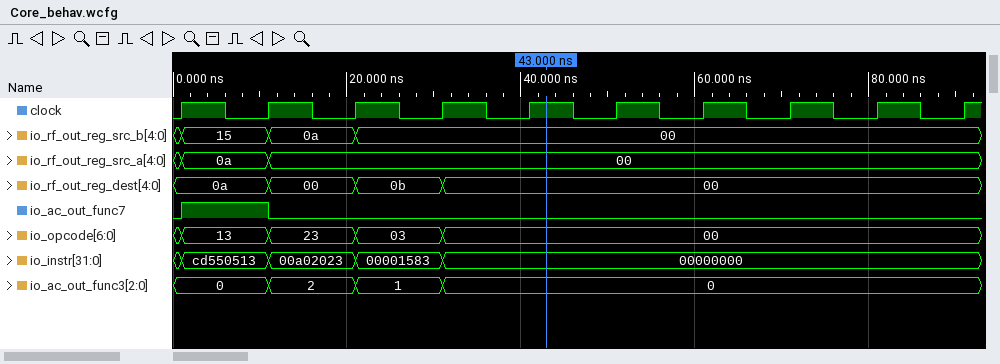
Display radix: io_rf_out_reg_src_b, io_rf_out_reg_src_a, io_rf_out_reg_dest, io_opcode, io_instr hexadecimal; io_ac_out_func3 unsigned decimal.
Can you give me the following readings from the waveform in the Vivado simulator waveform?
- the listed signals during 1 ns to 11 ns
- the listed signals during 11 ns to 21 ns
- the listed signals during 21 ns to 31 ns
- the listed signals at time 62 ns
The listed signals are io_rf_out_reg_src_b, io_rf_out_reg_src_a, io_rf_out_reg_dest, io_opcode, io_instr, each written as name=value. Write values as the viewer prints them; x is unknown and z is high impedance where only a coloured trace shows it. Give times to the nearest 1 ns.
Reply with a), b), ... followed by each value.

a) io_rf_out_reg_src_b=15, io_rf_out_reg_src_a=0a, io_rf_out_reg_dest=0a, io_opcode=13, io_instr=cd550513
b) io_rf_out_reg_src_b=0a, io_rf_out_reg_src_a=00, io_rf_out_reg_dest=00, io_opcode=23, io_instr=00a02023
c) io_rf_out_reg_src_b=00, io_rf_out_reg_src_a=00, io_rf_out_reg_dest=0b, io_opcode=03, io_instr=00001583
d) io_rf_out_reg_src_b=00, io_rf_out_reg_src_a=00, io_rf_out_reg_dest=00, io_opcode=00, io_instr=00000000
